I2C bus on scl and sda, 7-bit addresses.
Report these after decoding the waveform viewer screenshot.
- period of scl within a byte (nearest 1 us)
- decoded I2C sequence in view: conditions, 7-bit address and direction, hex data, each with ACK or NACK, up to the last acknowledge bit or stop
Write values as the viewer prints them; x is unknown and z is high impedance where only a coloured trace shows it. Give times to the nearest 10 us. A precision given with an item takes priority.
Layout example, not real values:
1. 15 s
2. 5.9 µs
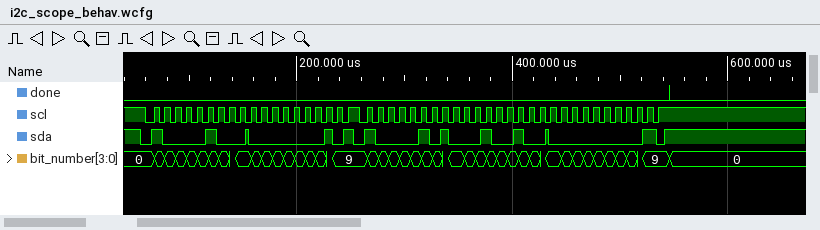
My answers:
1. 10 us
2. start, address 42 write ACK, 01 ACK, repeated start, address 42 read ACK, 24 ACK, 00 NACK, stop
